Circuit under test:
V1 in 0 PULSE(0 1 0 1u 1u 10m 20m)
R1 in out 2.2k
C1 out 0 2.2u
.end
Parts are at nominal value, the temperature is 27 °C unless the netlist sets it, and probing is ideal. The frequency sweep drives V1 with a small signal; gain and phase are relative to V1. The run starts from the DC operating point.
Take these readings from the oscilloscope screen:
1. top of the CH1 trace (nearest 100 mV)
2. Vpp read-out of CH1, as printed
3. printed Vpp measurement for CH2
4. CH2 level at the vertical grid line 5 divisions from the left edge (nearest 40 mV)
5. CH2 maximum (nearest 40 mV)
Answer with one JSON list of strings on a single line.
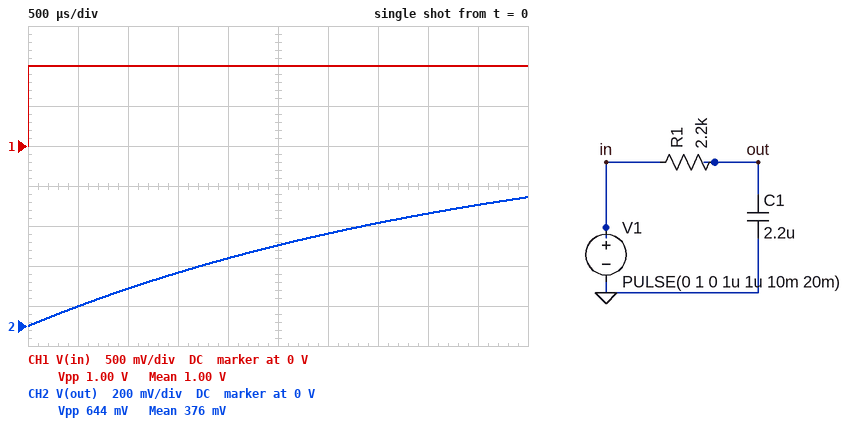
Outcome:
["1.0 V", "1.00 V", "644 mV", "400 mV", "640 mV"]
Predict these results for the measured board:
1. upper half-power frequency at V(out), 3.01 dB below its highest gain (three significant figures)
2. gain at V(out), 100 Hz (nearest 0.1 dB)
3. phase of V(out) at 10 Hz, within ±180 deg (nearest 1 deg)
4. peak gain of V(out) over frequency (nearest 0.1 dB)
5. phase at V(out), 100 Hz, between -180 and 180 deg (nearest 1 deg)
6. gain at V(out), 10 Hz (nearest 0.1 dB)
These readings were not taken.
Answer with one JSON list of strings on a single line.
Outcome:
["32.9 Hz", "-10.1 dB", "-17 deg", "0 dB", "-72 deg", "-0.4 dB"]
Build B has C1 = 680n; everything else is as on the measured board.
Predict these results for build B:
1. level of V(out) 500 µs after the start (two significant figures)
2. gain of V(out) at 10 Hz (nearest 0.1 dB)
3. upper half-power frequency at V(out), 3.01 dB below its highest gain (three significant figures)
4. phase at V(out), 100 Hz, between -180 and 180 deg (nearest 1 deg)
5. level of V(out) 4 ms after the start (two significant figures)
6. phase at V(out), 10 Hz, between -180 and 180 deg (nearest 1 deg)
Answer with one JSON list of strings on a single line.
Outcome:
["280 mV", "0 dB", "106 Hz", "-43 deg", "930 mV", "-5 deg"]
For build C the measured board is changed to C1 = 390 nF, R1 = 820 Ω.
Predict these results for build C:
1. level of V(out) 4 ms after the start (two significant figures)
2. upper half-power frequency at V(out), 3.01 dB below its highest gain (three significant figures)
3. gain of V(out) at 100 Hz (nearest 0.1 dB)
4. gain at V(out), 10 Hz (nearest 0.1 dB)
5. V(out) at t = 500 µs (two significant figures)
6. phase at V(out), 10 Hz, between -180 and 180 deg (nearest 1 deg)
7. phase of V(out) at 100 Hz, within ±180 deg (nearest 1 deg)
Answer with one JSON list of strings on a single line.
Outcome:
["1.0 V", "498 Hz", "-0.2 dB", "0 dB", "790 mV", "-1 deg", "-11 deg"]
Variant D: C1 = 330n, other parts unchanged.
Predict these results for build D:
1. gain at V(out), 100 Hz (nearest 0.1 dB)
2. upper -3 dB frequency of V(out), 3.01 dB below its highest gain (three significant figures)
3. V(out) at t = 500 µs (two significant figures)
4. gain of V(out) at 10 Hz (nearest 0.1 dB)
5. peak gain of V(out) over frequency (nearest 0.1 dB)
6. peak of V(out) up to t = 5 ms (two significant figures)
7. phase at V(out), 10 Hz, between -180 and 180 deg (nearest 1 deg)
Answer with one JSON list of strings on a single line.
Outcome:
["-0.8 dB", "219 Hz", "500 mV", "0 dB", "0 dB", "1.0 V", "-3 deg"]
